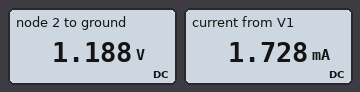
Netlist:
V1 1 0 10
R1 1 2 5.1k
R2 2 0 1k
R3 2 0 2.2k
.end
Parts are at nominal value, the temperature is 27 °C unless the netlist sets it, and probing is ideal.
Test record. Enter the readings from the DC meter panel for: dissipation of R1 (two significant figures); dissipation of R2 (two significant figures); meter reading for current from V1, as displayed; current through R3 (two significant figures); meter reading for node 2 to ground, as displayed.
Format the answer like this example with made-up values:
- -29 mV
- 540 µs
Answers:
- 15 mW
- 1.4 mW
- 1.728 mA
- 540 µA
- 1.188 V
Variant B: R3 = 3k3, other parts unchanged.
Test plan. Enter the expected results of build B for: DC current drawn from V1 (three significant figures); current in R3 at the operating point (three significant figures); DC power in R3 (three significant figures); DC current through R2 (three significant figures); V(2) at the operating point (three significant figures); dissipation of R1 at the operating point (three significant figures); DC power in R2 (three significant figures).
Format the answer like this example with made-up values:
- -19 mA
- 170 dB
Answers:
- 1.70 mA
- 396 µA
- 518 µW
- 1.31 mA
- 1.31 V
- 14.8 mW
- 1.71 mW
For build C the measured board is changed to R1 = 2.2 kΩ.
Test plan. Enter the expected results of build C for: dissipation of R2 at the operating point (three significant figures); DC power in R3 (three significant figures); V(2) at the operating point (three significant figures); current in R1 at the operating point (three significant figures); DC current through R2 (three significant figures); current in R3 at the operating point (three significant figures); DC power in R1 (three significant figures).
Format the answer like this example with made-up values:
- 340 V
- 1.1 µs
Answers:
- 5.67 mW
- 2.58 mW
- 2.38 V
- 3.46 mA
- 2.38 mA
- 1.08 mA
- 26.4 mW
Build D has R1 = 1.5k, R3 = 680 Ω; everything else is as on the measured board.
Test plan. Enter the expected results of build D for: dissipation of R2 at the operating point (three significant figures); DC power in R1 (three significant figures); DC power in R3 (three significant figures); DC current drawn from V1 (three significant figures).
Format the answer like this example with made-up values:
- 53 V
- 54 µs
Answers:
- 4.52 mW
- 41.3 mW
- 6.64 mW
- 5.25 mA
